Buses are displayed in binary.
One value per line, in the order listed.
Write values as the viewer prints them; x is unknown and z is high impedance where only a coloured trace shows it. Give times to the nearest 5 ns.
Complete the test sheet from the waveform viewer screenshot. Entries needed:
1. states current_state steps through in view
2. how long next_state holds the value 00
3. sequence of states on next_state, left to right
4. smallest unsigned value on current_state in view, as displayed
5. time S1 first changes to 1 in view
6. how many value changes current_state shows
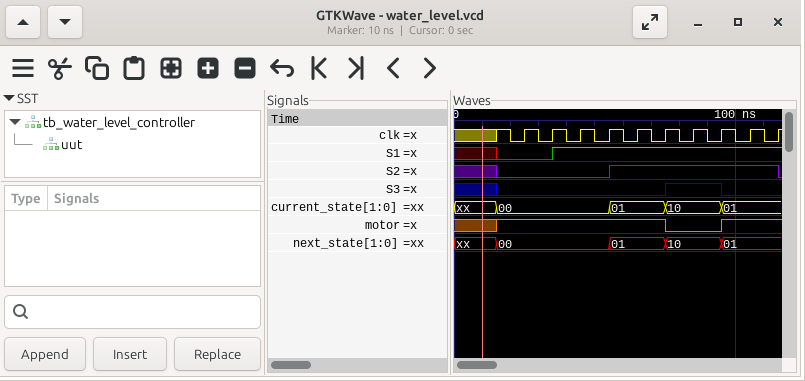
xx, 00, 01, 10, 01
40 ns
xx, 00, 01, 10, 01
00
35 ns
4
